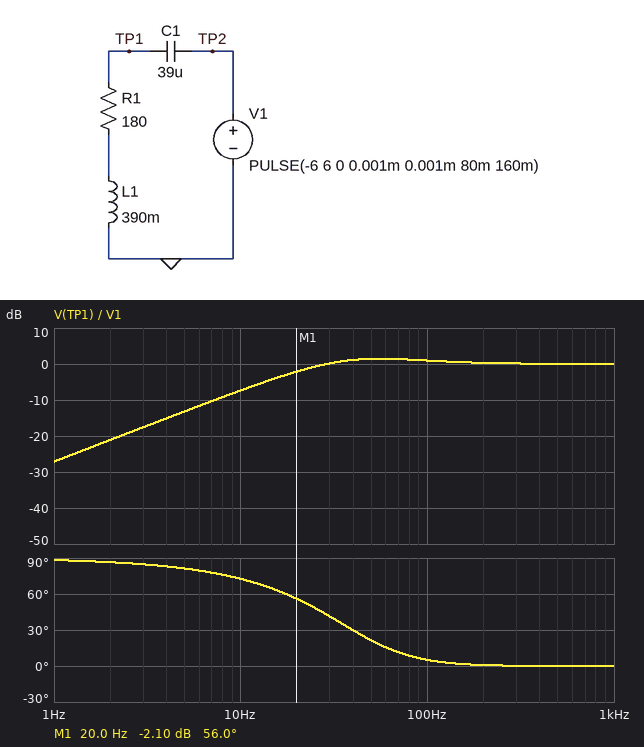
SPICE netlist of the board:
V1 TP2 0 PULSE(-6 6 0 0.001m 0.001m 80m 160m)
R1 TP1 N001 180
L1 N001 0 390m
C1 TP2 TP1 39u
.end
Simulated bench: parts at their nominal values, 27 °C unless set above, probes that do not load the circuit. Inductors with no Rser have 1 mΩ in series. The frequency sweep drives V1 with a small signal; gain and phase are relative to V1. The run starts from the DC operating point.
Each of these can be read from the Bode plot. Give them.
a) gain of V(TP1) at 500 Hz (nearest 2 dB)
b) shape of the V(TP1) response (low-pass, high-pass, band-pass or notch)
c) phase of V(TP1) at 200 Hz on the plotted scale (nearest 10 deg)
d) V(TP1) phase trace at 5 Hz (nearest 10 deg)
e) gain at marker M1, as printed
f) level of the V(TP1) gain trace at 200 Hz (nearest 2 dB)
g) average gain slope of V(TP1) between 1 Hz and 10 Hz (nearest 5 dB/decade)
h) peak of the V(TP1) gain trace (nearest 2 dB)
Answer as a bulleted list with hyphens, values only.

- 0 dB
- high-pass
- 0 deg
- 80 deg
- -2.10 dB
- 0 dB
- 20 dB/decade
- 2 dB
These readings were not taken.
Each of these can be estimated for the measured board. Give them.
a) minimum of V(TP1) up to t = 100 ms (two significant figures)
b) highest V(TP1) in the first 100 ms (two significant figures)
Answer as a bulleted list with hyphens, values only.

- -12 V
- 12 V
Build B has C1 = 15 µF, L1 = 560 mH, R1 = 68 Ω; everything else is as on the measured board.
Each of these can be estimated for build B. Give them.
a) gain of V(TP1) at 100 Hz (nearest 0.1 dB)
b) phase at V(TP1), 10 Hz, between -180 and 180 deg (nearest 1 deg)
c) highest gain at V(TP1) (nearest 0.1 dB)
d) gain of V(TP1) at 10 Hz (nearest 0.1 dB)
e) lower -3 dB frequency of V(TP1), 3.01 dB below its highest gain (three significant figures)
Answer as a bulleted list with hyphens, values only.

- 3.0 dB
- 114 deg
- 9.7 dB
- -22.6 dB
- 48.2 Hz
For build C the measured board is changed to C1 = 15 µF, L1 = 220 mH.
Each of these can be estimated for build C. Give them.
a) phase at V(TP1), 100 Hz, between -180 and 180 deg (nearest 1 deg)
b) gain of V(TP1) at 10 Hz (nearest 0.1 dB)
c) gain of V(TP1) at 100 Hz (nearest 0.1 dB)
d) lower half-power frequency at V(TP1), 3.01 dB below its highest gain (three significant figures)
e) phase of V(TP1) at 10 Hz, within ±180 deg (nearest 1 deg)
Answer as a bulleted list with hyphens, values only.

- 27 deg
- -15.4 dB
- 1.9 dB
- 53.2 Hz
- 85 deg
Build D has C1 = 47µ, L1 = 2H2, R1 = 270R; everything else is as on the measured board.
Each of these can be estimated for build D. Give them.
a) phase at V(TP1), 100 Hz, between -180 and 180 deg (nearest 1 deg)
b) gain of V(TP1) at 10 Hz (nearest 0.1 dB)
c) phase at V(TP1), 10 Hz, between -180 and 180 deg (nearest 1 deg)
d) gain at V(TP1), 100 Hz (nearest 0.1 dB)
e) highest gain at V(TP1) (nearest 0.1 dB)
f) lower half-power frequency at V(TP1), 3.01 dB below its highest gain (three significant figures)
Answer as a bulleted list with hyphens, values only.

- 0 deg
- -0.9 dB
- 64 deg
- 0.2 dB
- 2.5 dB
- 10.4 Hz
